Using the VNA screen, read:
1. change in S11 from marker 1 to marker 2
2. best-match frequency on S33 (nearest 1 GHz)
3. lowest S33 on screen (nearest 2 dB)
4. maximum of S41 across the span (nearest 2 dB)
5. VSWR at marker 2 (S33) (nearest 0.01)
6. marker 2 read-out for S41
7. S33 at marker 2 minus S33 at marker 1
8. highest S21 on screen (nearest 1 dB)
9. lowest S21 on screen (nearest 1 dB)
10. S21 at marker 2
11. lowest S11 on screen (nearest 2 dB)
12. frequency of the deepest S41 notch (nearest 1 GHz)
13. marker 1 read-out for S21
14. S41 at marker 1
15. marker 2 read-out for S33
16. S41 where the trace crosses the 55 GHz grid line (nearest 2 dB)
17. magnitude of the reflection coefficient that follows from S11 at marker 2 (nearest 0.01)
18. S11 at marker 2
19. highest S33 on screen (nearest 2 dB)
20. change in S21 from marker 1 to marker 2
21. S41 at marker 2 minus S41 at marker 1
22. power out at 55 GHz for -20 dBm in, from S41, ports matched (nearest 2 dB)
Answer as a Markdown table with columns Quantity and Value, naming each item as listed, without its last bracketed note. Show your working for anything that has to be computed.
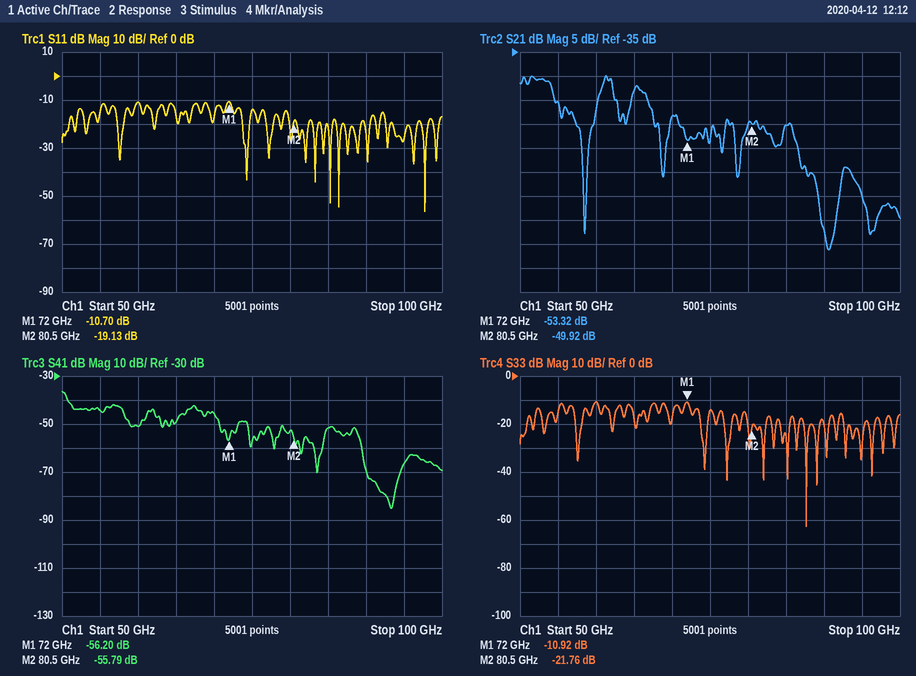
| Quantity | Value |
|---|---|
| change in S11 from marker 1 to marker 2 | -19.13 − (-10.7) = -8.43 dB |
| best-match frequency on S33 | 88 GHz |
| lowest S33 on screen | -62 dB |
| maximum of S41 across the span | -36 dB |
| VSWR at marker 2 (S33) | (1 + 0.0817)/(1 − 0.0817) ≈ 1.18 |
| marker 2 read-out for S41 | -55.79 dB |
| S33 at marker 2 minus S33 at marker 1 | -21.76 − (-10.92) = -10.84 dB |
| highest S21 on screen | -40 dB |
| lowest S21 on screen | -76 dB |
| S21 at marker 2 | -49.92 dB |
| lowest S11 on screen | -56 dB |
| frequency of the deepest S41 notch | 93 GHz |
| marker 1 read-out for S21 | -53.32 dB |
| S41 at marker 1 | -56.20 dB |
| marker 2 read-out for S33 | -21.76 dB |
| S41 where the trace crosses the 55 GHz grid line | -44 dB |
| magnitude of the reflection coefficient that follows from S11 at marker 2 | 10^(-19.13/20) ≈ 0.11 |
| S11 at marker 2 | -19.13 dB |
| highest S33 on screen | -10 dB |
| change in S21 from marker 1 to marker 2 | -49.92 − (-53.32) = 3.40 dB |
| S41 at marker 2 minus S41 at marker 1 | -55.79 − (-56.2) = 0.41 dB |
| power out at 55 GHz for -20 dBm in, from S41, ports matched | -20 dBm + (-44 dB) = -64 dBm |
